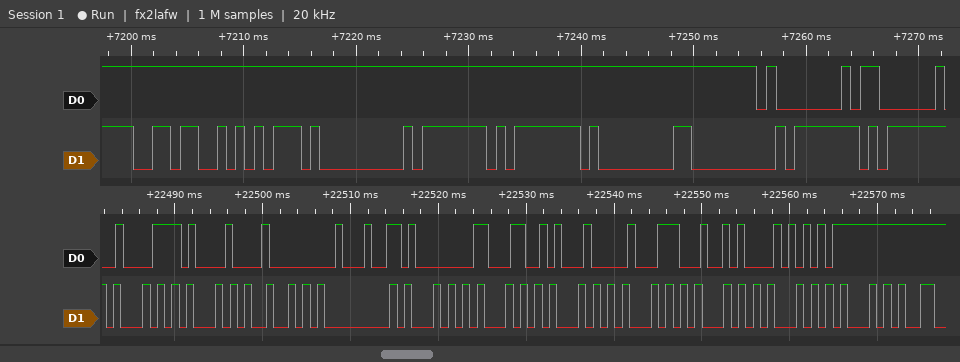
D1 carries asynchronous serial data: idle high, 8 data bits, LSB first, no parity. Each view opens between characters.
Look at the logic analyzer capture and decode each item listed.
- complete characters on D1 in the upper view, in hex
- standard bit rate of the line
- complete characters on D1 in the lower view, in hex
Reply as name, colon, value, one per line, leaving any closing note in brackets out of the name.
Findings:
complete characters on D1 in the upper view, in hex: 36, 75, 00, 7F, 7F, 80, 00, 7F
standard bit rate of the line: 1200 baud
complete characters on D1 in the lower view, in hex: 51, 51, 52, 00, 51, 51, 51, 51, 51, 51, 51
